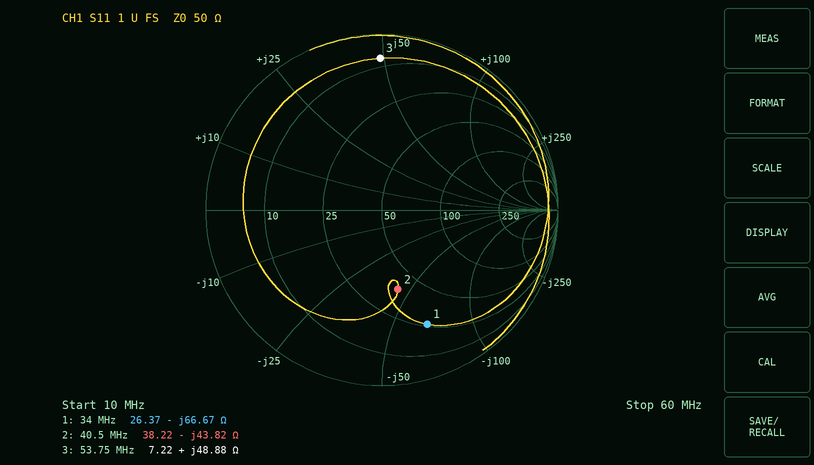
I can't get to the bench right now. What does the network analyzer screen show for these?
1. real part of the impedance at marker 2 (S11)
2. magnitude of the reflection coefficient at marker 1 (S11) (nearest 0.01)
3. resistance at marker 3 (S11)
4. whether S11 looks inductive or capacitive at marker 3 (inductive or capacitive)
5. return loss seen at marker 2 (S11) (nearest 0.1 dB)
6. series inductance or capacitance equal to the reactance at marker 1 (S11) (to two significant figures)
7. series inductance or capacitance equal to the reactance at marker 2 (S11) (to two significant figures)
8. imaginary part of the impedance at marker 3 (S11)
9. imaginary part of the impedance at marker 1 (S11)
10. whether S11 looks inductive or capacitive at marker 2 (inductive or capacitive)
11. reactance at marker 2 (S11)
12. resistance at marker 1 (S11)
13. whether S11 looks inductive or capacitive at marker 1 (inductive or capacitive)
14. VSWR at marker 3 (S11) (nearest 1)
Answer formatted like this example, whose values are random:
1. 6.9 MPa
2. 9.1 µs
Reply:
1. 38.22 Ω
2. 0.70
3. 7.22 Ω
4. inductive
5. 6.7 dB
6. 70 pF
7. 90 pF
8. +48.88 Ω
9. -66.67 Ω
10. capacitive
11. -43.82 Ω
12. 26.37 Ω
13. capacitive
14. 14
